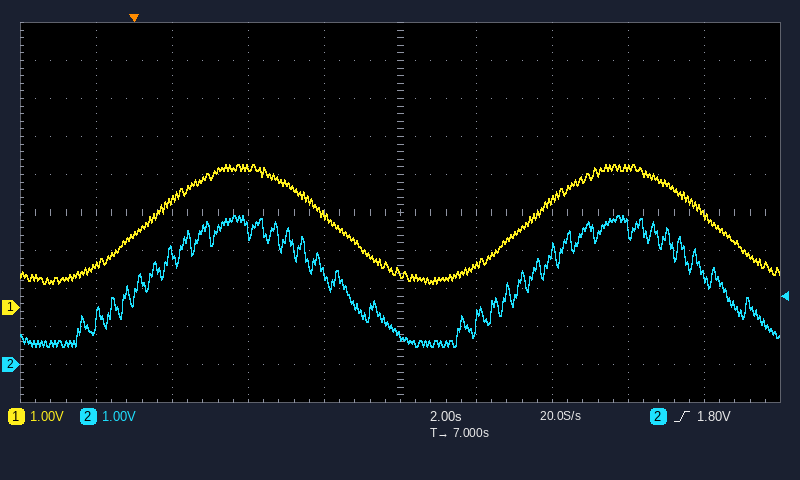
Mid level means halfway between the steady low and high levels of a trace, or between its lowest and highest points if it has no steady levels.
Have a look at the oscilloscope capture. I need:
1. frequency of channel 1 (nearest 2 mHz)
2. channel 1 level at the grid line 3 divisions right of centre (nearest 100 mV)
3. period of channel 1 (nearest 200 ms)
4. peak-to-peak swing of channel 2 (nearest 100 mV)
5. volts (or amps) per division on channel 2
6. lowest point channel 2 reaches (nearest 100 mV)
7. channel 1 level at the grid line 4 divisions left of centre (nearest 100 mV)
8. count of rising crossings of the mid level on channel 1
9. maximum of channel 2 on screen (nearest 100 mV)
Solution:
100 mHz
3.7 V
10.0 s
3.4 V
1 V
500 mV
1.1 V
2
3.9 V
